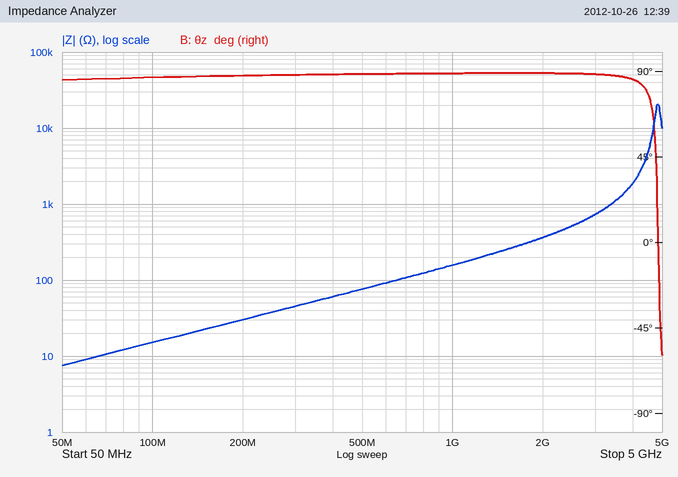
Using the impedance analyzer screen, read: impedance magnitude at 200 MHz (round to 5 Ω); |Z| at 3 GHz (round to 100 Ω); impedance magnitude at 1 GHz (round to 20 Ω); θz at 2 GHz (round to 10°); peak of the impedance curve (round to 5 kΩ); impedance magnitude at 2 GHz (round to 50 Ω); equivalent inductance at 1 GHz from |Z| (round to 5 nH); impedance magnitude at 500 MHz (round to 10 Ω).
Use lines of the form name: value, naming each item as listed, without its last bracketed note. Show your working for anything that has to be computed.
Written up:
impedance magnitude at 200 MHz: 30 Ω
|Z| at 3 GHz: 700 Ω
impedance magnitude at 1 GHz: 160 Ω
θz at 2 GHz: 90°
peak of the impedance curve: 20 kΩ
impedance magnitude at 2 GHz: 350 Ω
equivalent inductance at 1 GHz from |Z|: L = 160 Ω/(2π × 1 GHz) ≈ 25 nH
impedance magnitude at 500 MHz: 80 Ω
